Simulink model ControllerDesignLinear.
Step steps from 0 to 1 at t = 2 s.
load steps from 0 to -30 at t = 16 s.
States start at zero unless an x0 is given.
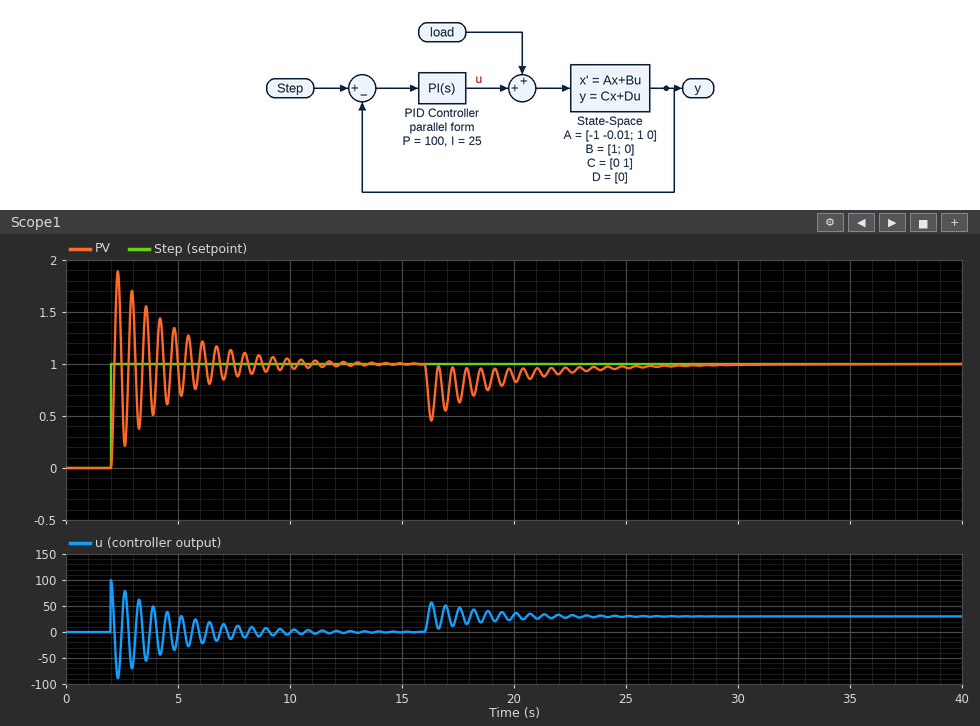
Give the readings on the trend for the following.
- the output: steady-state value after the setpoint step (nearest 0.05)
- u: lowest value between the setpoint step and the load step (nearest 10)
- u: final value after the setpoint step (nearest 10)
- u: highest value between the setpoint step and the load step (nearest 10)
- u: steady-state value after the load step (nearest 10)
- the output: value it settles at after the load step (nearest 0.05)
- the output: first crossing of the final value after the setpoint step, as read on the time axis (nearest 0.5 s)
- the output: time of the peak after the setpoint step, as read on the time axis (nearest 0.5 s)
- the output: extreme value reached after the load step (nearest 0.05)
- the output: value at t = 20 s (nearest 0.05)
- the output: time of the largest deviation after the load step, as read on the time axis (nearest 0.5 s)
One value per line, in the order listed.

1.00
-90
0
100
30
1.00
2.0 s
2.5 s
0.45
0.85
16.5 s
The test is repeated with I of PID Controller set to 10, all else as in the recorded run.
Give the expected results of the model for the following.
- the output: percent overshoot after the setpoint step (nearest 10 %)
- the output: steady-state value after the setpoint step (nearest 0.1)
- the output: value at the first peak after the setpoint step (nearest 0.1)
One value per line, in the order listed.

90 %
1.0
1.9
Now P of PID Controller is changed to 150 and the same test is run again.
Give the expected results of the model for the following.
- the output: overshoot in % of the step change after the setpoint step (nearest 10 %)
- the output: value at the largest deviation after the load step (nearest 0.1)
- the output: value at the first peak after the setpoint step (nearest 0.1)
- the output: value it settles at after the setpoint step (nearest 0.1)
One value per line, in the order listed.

90 %
0.6
1.9
1.0
